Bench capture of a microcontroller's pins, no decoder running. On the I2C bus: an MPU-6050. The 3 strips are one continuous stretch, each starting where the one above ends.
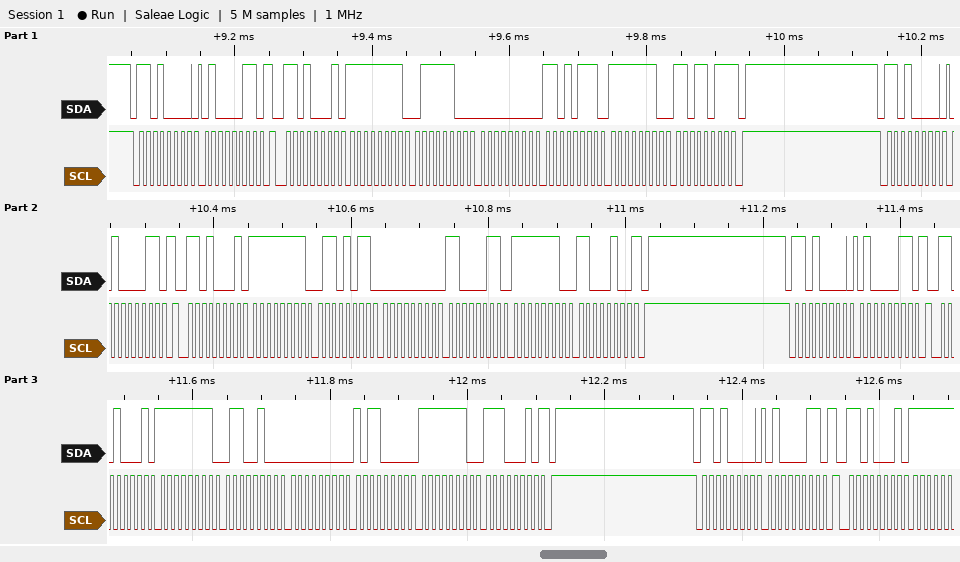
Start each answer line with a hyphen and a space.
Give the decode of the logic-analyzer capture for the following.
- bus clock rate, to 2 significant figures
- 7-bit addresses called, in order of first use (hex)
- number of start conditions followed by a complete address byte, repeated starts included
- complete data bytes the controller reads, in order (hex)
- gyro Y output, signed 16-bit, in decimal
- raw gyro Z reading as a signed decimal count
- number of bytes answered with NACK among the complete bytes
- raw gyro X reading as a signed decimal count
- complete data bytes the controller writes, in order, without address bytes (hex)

- 100 kHz
- 0x68
- 8
- FF 7C 00 D7 FE DB FF 6B 00 C3 FE C4 FF 64 00 B0 FE E2
- 215
- -293
- 3
- -132
- 43 43 43 43
